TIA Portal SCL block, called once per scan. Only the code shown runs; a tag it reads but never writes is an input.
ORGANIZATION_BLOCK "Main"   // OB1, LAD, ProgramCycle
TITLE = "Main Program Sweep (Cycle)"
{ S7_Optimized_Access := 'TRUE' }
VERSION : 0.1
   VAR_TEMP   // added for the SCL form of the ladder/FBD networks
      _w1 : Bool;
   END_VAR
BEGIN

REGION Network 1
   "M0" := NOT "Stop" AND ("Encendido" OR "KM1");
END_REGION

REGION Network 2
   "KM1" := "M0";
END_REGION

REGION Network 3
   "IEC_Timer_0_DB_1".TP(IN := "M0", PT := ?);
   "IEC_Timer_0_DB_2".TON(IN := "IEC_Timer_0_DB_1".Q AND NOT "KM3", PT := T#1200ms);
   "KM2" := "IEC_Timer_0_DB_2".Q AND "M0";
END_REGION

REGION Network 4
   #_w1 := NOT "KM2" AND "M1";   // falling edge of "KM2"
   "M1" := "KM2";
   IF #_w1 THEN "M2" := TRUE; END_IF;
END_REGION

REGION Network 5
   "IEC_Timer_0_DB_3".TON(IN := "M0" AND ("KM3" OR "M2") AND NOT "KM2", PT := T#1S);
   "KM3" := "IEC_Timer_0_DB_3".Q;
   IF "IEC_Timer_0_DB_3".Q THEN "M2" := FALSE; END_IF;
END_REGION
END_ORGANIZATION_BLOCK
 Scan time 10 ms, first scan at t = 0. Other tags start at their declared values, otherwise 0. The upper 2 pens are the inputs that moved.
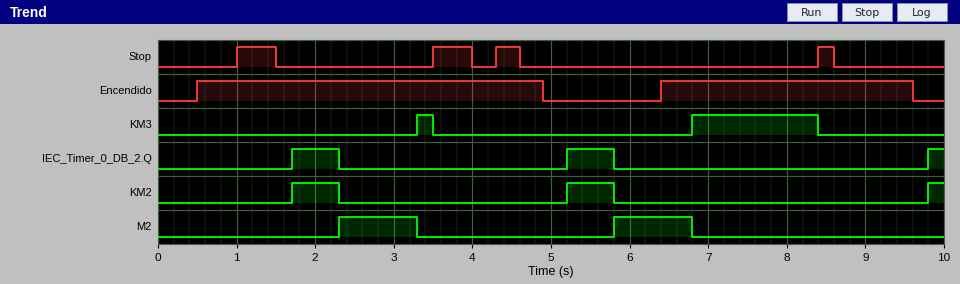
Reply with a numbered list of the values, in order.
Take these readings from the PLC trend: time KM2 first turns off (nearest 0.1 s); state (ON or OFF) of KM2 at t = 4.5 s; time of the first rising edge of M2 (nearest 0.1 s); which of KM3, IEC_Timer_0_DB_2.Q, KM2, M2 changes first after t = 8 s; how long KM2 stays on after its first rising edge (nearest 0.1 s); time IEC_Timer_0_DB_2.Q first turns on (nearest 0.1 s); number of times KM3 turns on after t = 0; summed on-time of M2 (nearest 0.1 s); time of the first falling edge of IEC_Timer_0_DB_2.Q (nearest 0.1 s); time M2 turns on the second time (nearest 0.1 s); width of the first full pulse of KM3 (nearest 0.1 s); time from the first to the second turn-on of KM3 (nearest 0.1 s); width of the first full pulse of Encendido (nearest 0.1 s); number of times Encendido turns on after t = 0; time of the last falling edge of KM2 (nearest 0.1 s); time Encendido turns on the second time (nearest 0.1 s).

1. 2.3 s
2. OFF
3. 2.3 s
4. KM3
5. 0.6 s
6. 1.7 s
7. 2
8. 2.0 s
9. 2.3 s
10. 5.8 s
11. 0.2 s
12. 3.5 s
13. 4.4 s
14. 2
15. 5.8 s
16. 6.4 s
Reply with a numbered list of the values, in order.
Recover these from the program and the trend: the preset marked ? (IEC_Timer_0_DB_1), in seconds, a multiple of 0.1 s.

1. 1.8 s
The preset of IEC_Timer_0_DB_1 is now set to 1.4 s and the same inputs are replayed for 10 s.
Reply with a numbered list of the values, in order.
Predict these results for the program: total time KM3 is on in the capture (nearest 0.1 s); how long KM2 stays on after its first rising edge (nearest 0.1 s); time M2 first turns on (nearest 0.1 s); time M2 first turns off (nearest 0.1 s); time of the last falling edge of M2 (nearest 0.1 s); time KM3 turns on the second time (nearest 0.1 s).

1. 2.6 s
2. 0.2 s
3. 1.9 s
4. 2.9 s
5. 6.4 s
6. 6.4 s
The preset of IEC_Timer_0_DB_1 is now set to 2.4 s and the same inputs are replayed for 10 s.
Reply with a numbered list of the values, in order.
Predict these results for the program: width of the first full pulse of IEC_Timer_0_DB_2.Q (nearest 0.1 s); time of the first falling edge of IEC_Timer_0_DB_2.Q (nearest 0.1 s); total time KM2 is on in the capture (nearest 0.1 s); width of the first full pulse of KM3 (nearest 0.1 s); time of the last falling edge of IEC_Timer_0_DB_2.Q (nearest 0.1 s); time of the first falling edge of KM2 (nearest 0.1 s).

1. 1.2 s
2. 2.9 s
3. 2.6 s
4. 1.0 s
5. 6.4 s
6. 2.9 s
